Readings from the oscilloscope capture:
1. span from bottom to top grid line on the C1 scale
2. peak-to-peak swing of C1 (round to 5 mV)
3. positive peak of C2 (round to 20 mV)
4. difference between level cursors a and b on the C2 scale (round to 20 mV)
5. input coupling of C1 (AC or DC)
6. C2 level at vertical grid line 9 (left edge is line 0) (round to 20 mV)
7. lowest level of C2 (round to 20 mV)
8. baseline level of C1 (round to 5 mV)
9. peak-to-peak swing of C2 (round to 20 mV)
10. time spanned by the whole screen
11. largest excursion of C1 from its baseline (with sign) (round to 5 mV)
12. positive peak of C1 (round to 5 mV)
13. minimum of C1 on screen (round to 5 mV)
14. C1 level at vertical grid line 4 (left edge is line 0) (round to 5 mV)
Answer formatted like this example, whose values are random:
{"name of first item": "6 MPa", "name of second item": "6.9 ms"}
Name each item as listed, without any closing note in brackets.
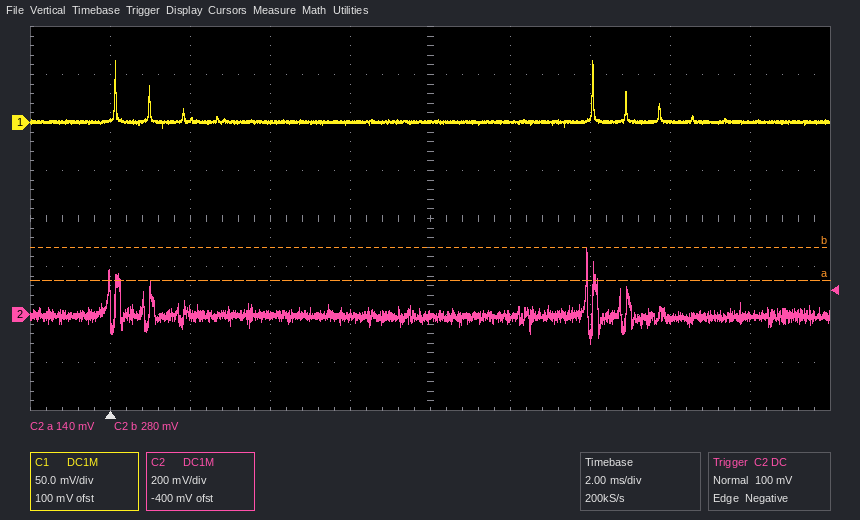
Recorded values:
{"span from bottom to top grid line on the C1 scale": "400 mV", "peak-to-peak swing of C1": "70 mV", "positive peak of C2": "280 mV", "difference between level cursors a and b on the C2 scale": "140 mV", "input coupling of C1": "DC", "C2 level at vertical grid line 9 (left edge is line 0)": "0 mV", "lowest level of C2": "-120 mV", "baseline level of C1": "0 mV", "peak-to-peak swing of C2": "400 mV", "time spanned by the whole screen": "20 ms", "largest excursion of C1 from its baseline (with sign)": "+65 mV", "positive peak of C1": "65 mV", "minimum of C1 on screen": "-5 mV", "C1 level at vertical grid line 4 (left edge is line 0)": "0 mV"}
